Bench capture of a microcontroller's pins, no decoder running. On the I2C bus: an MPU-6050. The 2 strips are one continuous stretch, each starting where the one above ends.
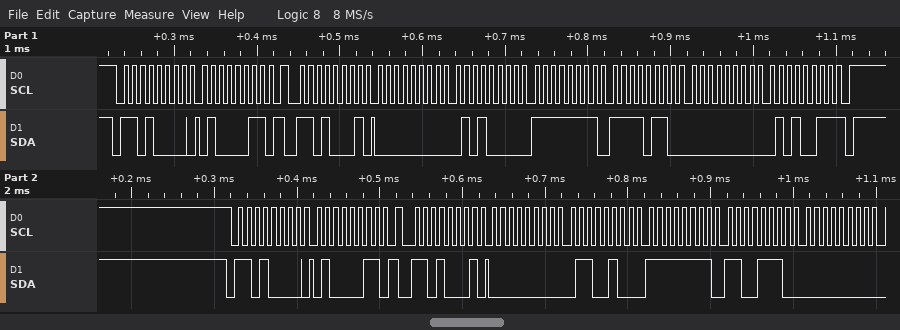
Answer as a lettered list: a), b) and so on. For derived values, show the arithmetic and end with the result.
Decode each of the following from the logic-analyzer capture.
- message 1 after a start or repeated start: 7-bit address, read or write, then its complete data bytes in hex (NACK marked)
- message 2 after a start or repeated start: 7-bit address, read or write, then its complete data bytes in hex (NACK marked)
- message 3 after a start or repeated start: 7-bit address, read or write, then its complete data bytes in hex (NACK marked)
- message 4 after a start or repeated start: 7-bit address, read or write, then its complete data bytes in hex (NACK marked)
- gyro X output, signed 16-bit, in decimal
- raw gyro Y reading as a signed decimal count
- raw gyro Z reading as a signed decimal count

a) 0x68 write: 43
b) 0x68 read: 00 50 FF F6 00 53 NACK
c) 0x68 write: 43
d) 0x68 read: 00 64 FF CE 00
e) 0x0050 = 80
f) 0xFFF6 = -10
g) 0x0053 = 83
